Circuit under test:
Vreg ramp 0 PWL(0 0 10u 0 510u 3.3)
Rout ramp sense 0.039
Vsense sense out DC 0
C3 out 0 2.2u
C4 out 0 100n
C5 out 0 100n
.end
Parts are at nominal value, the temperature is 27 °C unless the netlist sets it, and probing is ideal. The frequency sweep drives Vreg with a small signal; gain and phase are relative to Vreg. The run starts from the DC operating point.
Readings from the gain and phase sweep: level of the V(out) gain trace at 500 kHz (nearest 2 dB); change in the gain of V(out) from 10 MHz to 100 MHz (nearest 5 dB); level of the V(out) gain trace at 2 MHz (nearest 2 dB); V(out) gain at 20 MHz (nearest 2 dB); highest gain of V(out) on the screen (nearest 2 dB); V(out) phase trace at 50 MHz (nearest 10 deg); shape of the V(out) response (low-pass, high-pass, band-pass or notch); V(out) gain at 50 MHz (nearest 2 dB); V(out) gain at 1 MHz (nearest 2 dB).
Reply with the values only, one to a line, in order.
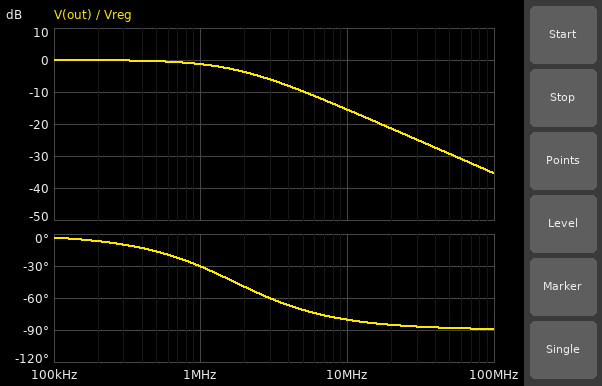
0 dB
-20 dB
-4 dB
-22 dB
0 dB
-90 deg
low-pass
-30 dB
-2 dB
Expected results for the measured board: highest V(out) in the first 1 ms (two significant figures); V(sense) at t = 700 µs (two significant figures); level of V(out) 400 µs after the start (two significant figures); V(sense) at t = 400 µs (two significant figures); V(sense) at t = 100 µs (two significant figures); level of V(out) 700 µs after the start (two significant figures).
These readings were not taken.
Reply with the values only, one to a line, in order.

3.3 V
3.3 V
2.6 V
2.6 V
590 mV
3.3 V
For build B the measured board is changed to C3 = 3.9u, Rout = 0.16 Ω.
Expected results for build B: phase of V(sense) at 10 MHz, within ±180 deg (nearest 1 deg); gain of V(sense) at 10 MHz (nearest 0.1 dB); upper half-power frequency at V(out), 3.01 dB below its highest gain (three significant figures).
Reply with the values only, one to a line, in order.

-89 deg
-32.3 dB
243 kHz
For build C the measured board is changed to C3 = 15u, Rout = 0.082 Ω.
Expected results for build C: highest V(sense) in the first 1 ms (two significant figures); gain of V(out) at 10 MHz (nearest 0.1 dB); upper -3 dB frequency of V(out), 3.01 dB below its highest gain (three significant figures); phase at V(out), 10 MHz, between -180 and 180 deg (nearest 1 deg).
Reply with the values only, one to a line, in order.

3.3 V
-37.9 dB
128 kHz
-89 deg
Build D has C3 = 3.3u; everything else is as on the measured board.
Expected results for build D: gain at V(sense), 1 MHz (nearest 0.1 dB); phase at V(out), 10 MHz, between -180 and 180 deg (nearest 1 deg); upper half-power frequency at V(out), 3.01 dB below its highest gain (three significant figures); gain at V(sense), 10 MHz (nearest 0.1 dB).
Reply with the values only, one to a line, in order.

-2.4 dB
-83 deg
1.17 MHz
-18.7 dB
